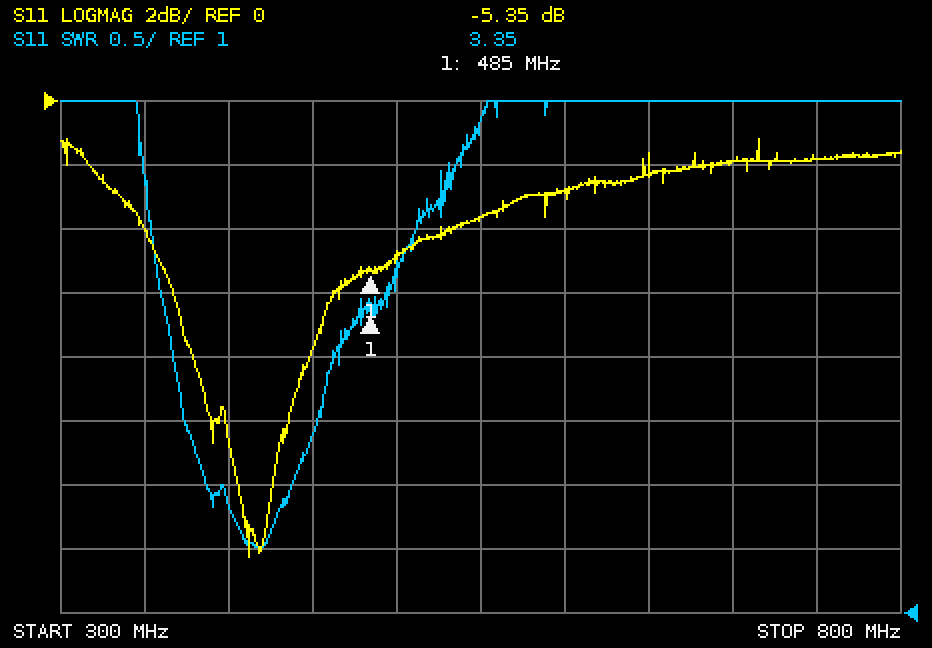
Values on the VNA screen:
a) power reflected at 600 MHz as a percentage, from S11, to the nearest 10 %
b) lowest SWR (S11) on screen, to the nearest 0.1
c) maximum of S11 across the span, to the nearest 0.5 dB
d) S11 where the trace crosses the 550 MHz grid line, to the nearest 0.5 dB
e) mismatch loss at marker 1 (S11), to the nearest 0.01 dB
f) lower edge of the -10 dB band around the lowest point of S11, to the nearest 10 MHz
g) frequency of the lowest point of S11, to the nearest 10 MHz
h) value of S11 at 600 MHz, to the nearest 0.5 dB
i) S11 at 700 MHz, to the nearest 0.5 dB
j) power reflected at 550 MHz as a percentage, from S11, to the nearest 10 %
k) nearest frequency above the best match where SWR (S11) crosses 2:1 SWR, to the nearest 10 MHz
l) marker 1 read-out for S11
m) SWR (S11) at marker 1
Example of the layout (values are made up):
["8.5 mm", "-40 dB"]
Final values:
["50 %", "1.5", "-1.0 dB", "-3.5 dB", "1.50 dB", "400 MHz", "410 MHz", "-3.0 dB", "-2.0 dB", "40 %", "440 MHz", "-5.35 dB", "3.35"]
